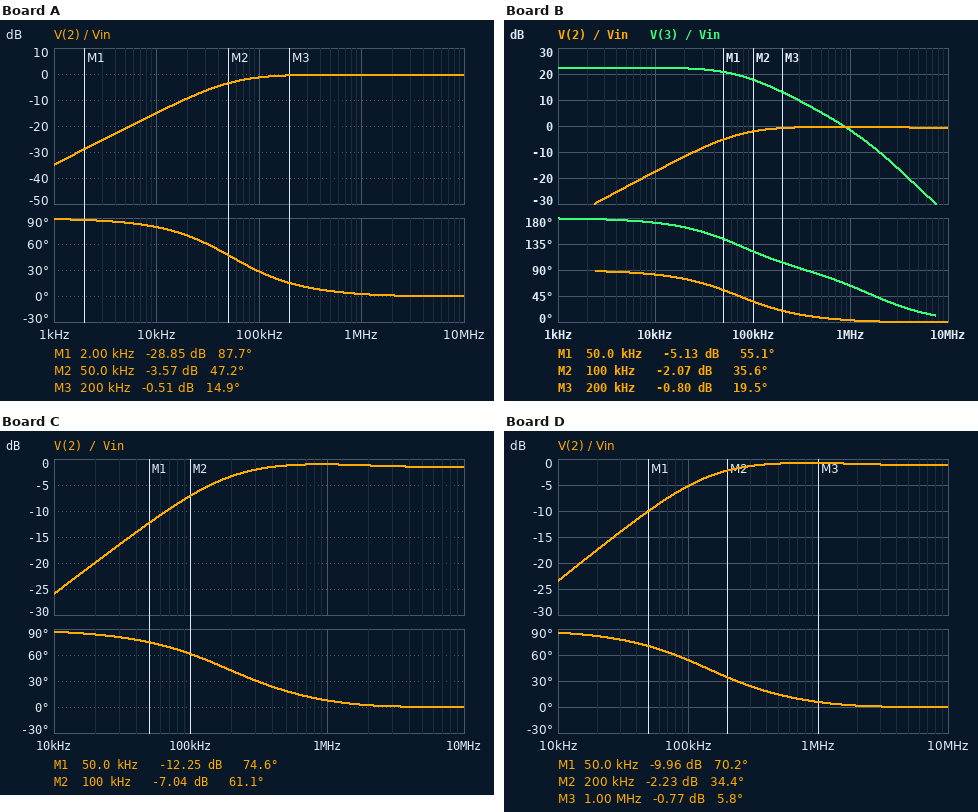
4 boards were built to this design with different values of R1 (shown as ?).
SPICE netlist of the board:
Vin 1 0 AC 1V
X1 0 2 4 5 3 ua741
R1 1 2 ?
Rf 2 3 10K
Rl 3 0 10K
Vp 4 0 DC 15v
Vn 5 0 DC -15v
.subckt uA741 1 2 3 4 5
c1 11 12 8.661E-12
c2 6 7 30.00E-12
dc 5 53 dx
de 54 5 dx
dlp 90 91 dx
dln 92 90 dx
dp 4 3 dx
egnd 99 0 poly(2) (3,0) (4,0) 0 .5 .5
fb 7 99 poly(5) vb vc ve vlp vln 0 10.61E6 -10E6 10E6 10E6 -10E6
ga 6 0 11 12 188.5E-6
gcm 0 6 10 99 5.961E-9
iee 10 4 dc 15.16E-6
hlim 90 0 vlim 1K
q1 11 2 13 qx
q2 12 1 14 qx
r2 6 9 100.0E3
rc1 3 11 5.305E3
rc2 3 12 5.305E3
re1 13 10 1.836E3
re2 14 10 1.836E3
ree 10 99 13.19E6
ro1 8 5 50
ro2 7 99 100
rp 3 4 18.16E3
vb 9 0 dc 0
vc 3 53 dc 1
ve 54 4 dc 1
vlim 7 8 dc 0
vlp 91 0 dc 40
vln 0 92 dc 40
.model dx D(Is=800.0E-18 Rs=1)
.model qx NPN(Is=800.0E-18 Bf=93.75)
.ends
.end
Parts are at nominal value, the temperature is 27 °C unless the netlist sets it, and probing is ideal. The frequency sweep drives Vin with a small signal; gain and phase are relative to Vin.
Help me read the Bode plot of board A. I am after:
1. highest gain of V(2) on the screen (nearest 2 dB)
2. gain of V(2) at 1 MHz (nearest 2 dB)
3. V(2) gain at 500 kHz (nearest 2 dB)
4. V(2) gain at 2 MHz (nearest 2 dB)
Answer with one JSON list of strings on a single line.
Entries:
["0 dB", "0 dB", "0 dB", "0 dB"]
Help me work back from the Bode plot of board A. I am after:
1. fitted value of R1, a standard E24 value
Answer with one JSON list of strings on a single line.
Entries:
["560 Ω"]
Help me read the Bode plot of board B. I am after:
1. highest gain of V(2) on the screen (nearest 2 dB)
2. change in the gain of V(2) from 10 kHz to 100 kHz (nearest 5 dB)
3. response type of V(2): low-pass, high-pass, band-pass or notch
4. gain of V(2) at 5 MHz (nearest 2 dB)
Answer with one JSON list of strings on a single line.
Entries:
["0 dB", "15 dB", "high-pass", "0 dB"]
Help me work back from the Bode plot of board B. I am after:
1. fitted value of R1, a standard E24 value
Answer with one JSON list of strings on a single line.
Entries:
["750 Ω"]
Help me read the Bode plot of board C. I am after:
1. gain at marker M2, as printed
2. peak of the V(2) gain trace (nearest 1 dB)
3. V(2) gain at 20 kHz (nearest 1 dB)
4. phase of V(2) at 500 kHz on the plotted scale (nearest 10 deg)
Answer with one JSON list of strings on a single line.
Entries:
["-7.04 dB", "-1 dB", "-20 dB", "20 deg"]
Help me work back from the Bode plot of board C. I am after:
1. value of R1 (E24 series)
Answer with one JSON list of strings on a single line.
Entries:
["2 kΩ"]
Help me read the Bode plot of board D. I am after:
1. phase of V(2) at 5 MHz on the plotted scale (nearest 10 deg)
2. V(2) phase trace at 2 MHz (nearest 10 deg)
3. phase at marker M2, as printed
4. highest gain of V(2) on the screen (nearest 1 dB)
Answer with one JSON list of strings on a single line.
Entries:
["0 deg", "0 deg", "34.4 deg", "-1 dB"]
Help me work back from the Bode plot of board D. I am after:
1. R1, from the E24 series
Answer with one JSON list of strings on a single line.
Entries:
["1.5 kΩ"]
